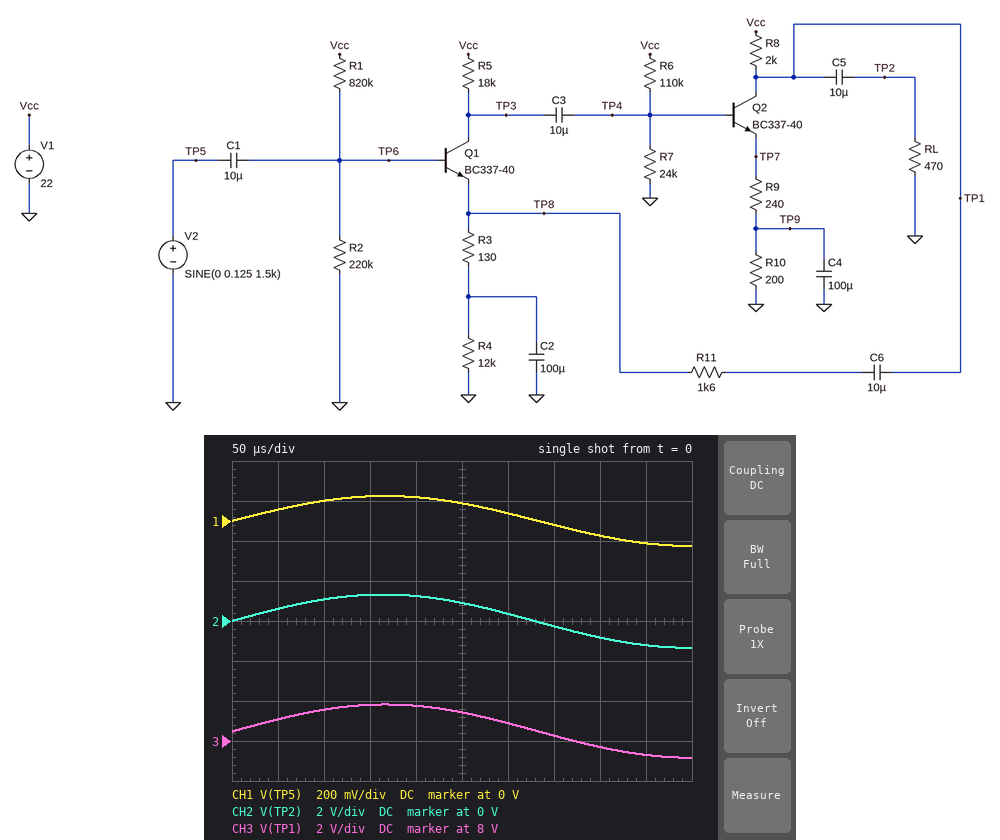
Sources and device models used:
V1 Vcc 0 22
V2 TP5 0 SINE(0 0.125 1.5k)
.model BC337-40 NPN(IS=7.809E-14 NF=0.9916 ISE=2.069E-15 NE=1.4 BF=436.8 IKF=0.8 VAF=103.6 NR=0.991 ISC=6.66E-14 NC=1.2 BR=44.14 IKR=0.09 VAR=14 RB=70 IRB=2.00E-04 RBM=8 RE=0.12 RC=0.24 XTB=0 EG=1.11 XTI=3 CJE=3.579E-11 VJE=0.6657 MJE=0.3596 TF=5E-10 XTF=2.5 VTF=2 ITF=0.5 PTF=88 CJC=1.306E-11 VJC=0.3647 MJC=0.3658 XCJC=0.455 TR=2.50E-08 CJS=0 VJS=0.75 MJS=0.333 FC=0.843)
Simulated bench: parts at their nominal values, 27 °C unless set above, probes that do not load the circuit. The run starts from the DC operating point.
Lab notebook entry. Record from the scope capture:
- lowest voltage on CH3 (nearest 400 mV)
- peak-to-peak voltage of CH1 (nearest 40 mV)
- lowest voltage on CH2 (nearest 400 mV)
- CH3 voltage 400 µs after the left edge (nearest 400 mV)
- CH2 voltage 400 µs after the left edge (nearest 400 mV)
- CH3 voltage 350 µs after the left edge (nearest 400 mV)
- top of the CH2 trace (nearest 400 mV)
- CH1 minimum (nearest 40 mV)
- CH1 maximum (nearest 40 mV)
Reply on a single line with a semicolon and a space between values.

7.2 V; 240 mV; -1.2 V; 7.6 V; -800 mV; 8.4 V; 1.2 V; -120 mV; 120 mV
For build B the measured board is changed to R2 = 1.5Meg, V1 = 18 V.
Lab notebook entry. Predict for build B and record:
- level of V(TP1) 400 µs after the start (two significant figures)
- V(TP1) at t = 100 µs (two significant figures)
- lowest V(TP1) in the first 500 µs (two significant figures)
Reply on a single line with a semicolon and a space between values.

6.6 V; 7.4 V; 6.0 V
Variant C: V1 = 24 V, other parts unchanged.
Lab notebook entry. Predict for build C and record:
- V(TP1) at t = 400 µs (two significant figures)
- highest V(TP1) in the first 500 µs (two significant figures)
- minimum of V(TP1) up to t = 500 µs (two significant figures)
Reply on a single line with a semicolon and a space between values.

8.2 V; 10 V; 7.7 V
